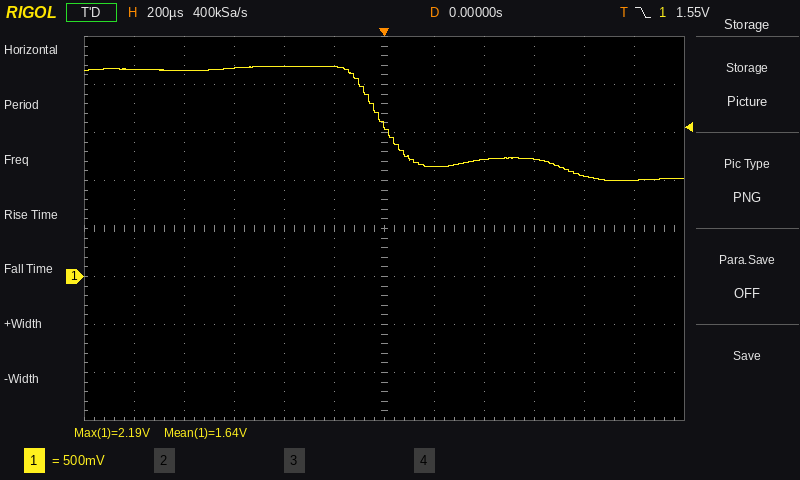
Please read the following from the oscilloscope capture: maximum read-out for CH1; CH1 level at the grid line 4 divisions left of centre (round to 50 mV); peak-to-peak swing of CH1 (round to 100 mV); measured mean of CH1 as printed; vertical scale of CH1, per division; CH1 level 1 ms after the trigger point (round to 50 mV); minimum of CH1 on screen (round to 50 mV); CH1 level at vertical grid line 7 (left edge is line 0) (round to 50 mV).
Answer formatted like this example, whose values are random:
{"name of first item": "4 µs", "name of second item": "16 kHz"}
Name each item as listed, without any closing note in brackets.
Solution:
{"maximum read-out for CH1": "2.19 V", "CH1 level at the grid line 4 divisions left of centre": "2.15 V", "peak-to-peak swing of CH1": "1.20 V", "measured mean of CH1 as printed": "1.64 V", "vertical scale of CH1, per division": "500 mV", "CH1 level 1 ms after the trigger point": "1.00 V", "minimum of CH1 on screen": "1.00 V", "CH1 level at vertical grid line 7 (left edge is line 0)": "1.15 V"}
